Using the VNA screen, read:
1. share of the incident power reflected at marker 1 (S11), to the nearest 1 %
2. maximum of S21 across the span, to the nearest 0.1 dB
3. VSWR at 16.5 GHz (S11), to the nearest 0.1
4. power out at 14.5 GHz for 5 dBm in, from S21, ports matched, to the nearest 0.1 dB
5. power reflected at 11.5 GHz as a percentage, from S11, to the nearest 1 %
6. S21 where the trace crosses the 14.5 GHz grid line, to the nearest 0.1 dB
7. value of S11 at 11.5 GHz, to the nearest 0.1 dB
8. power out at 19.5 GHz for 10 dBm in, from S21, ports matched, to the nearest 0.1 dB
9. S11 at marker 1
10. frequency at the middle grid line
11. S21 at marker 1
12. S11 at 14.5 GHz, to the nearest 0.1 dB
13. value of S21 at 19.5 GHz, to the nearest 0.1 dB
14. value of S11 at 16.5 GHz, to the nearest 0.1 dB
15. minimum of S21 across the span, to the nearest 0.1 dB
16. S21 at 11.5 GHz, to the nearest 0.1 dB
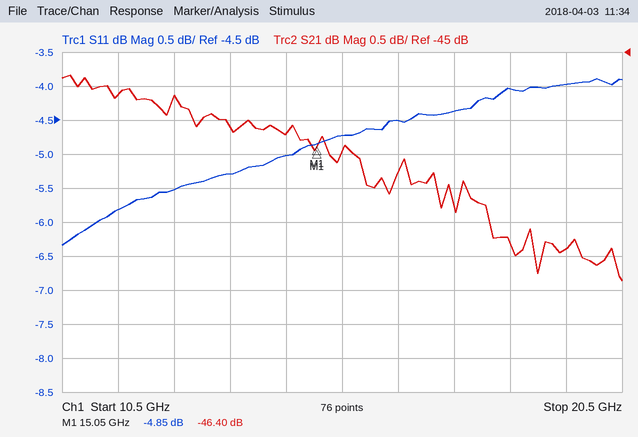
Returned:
33 %
-45.3 dB
3.9
-41.2 dBm
26 %
-46.2 dB
-5.8 dB
-37.9 dBm
-4.85 dB
15.5 GHz
-46.40 dB
-5.0 dB
-47.9 dB
-4.5 dB
-48.4 dB
-45.6 dB
